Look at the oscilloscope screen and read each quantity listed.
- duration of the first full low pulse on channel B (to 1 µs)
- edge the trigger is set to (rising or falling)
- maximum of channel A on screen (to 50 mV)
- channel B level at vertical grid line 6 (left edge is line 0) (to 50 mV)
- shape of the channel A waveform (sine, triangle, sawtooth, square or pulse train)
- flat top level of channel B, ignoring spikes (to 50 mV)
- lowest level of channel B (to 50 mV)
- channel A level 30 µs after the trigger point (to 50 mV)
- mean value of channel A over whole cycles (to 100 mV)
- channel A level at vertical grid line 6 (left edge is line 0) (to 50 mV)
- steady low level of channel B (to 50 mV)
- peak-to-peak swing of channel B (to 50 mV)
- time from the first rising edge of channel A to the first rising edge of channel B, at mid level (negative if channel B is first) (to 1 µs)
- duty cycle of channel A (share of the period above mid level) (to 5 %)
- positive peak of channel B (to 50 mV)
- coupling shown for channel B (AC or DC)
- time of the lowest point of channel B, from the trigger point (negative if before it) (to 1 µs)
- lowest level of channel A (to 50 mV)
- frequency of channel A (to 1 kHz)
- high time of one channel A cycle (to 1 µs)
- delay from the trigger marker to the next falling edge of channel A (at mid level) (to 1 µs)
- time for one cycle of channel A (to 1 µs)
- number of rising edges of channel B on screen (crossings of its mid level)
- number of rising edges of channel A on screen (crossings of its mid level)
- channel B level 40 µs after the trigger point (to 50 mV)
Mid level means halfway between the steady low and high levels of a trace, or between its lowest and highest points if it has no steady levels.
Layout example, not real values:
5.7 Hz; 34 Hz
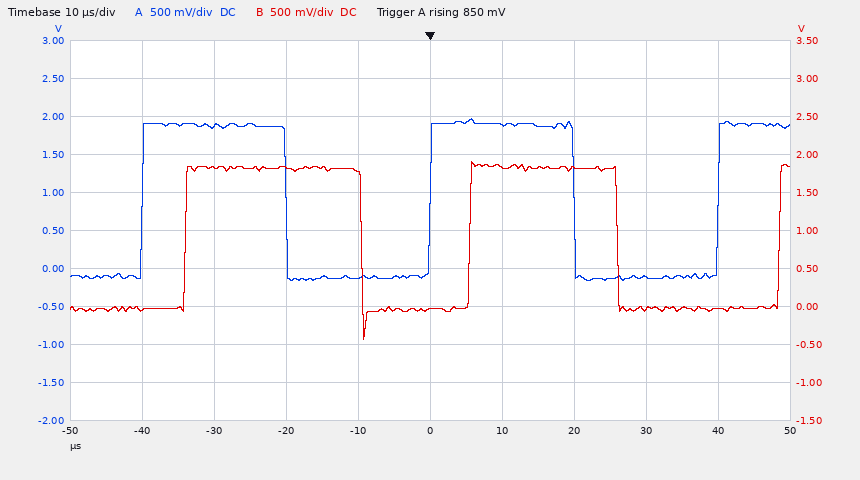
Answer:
15 µs; rising; 1.95 V; 1.85 V; square; 1.80 V; -450 mV; -100 mV; 900 mV; 1.90 V; -50 mV; 2.35 V; +6 µs; 50 %; 1.90 V; DC; -9 µs; -150 mV; 25 kHz; 20 µs; 20 µs; 40 µs; 3; 3; -50 mV
